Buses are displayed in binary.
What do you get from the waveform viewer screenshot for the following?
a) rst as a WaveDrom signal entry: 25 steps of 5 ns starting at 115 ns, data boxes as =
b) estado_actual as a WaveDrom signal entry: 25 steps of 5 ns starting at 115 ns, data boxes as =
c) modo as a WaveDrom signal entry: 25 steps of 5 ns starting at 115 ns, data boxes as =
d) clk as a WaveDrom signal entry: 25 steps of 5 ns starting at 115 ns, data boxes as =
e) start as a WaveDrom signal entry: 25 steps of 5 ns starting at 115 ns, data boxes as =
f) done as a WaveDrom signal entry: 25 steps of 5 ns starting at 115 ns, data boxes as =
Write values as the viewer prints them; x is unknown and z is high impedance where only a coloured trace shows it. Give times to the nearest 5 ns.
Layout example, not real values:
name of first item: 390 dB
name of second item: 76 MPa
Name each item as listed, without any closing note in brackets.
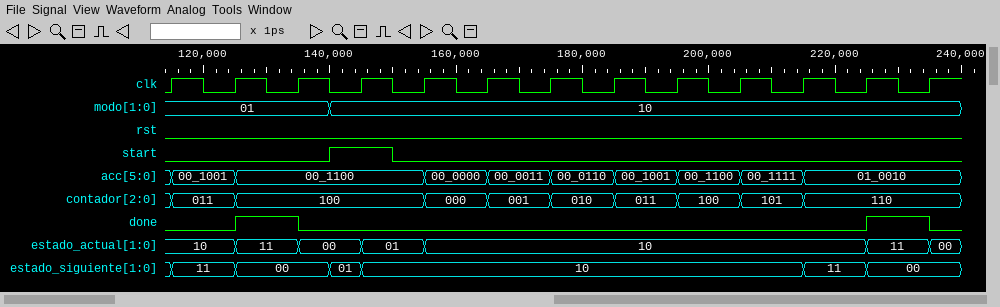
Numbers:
rst as a WaveDrom signal entry: 25 steps of 5 ns starting at 115 ns, data boxes as =: {name: 'rst', wave: '0........................'}
estado_actual as a WaveDrom signal entry: 25 steps of 5 ns starting at 115 ns, data boxes as =: {name: 'estado_actual', wave: '=.=.=.=.=.............=.=', data: '10 11 00 01 10 11 00'}
modo as a WaveDrom signal entry: 25 steps of 5 ns starting at 115 ns, data boxes as =: {name: 'modo', wave: '=....=...................', data: '01 10'}
clk as a WaveDrom signal entry: 25 steps of 5 ns starting at 115 ns, data boxes as =: {name: 'clk', wave: '1010101010101010101010101'}
start as a WaveDrom signal entry: 25 steps of 5 ns starting at 115 ns, data boxes as =: {name: 'start', wave: '0....1.0.................'}
done as a WaveDrom signal entry: 25 steps of 5 ns starting at 115 ns, data boxes as =: {name: 'done', wave: '0.1.0.................1.0'}
